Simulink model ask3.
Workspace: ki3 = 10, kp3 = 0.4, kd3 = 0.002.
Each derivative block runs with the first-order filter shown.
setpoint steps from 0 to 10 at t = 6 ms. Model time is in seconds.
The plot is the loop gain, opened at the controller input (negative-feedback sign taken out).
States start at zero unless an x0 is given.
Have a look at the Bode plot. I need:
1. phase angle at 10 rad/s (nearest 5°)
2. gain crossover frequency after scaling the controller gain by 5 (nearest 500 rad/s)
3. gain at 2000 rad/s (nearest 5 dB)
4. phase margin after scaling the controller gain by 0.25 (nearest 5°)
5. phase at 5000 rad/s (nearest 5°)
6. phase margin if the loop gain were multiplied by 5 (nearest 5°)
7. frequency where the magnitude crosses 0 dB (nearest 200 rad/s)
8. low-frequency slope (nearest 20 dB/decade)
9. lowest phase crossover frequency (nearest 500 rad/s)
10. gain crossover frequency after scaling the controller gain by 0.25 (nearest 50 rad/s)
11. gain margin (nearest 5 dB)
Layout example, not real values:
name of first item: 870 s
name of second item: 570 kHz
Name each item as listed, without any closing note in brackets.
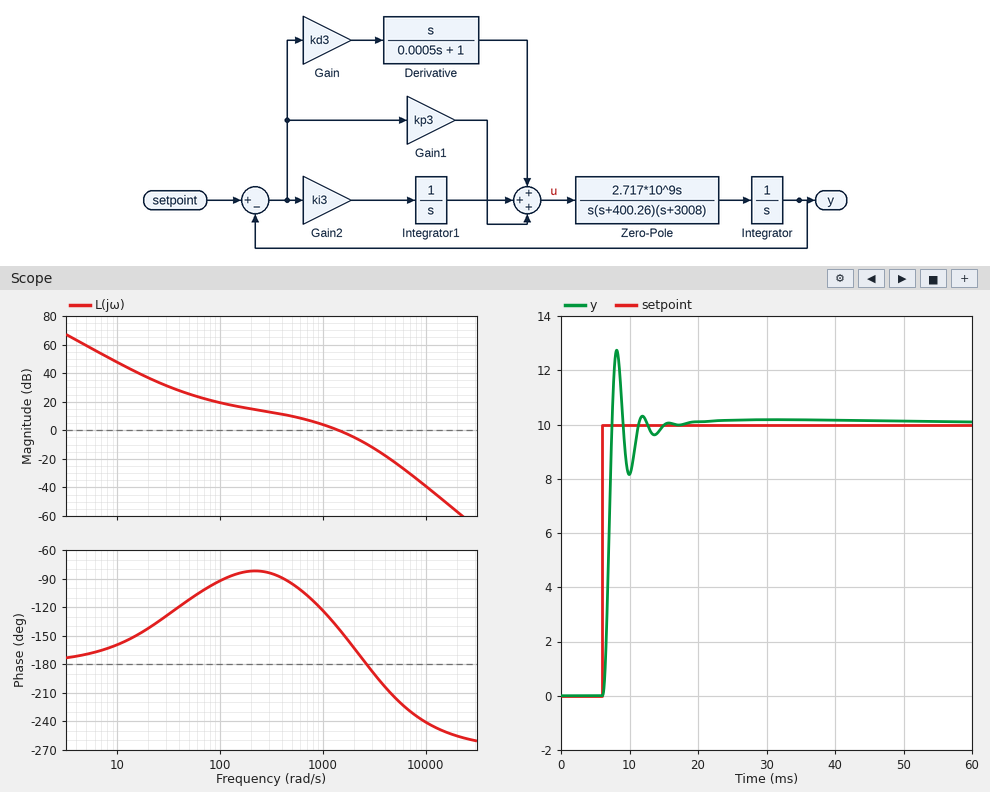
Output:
phase angle at 10 rad/s: -160°
gain crossover frequency after scaling the controller gain by 5: 3500 rad/s
gain at 2000 rad/s: -5 dB
phase margin after scaling the controller gain by 0.25: 95°
phase at 5000 rad/s: -215°
phase margin if the loop gain were multiplied by 5: -15°
frequency where the magnitude crosses 0 dB: 1400 rad/s
low-frequency slope: -40 dB/decade
lowest phase crossover frequency: 2500 rad/s
gain crossover frequency after scaling the controller gain by 0.25: 350 rad/s
gain margin: 10 dB
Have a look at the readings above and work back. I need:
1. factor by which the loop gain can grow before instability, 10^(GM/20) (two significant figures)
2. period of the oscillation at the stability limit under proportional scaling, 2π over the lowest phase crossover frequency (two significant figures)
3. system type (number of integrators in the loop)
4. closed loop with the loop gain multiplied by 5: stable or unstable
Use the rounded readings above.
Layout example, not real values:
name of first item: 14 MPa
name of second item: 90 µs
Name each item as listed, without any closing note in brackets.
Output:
factor by which the loop gain can grow before instability, 10^(GM/20): 3.2
period of the oscillation at the stability limit under proportional scaling, 2π over the lowest phase crossover frequency: 0.0025 s
system type: 2
closed loop with the loop gain multiplied by 5: stable or unstable: unstable
